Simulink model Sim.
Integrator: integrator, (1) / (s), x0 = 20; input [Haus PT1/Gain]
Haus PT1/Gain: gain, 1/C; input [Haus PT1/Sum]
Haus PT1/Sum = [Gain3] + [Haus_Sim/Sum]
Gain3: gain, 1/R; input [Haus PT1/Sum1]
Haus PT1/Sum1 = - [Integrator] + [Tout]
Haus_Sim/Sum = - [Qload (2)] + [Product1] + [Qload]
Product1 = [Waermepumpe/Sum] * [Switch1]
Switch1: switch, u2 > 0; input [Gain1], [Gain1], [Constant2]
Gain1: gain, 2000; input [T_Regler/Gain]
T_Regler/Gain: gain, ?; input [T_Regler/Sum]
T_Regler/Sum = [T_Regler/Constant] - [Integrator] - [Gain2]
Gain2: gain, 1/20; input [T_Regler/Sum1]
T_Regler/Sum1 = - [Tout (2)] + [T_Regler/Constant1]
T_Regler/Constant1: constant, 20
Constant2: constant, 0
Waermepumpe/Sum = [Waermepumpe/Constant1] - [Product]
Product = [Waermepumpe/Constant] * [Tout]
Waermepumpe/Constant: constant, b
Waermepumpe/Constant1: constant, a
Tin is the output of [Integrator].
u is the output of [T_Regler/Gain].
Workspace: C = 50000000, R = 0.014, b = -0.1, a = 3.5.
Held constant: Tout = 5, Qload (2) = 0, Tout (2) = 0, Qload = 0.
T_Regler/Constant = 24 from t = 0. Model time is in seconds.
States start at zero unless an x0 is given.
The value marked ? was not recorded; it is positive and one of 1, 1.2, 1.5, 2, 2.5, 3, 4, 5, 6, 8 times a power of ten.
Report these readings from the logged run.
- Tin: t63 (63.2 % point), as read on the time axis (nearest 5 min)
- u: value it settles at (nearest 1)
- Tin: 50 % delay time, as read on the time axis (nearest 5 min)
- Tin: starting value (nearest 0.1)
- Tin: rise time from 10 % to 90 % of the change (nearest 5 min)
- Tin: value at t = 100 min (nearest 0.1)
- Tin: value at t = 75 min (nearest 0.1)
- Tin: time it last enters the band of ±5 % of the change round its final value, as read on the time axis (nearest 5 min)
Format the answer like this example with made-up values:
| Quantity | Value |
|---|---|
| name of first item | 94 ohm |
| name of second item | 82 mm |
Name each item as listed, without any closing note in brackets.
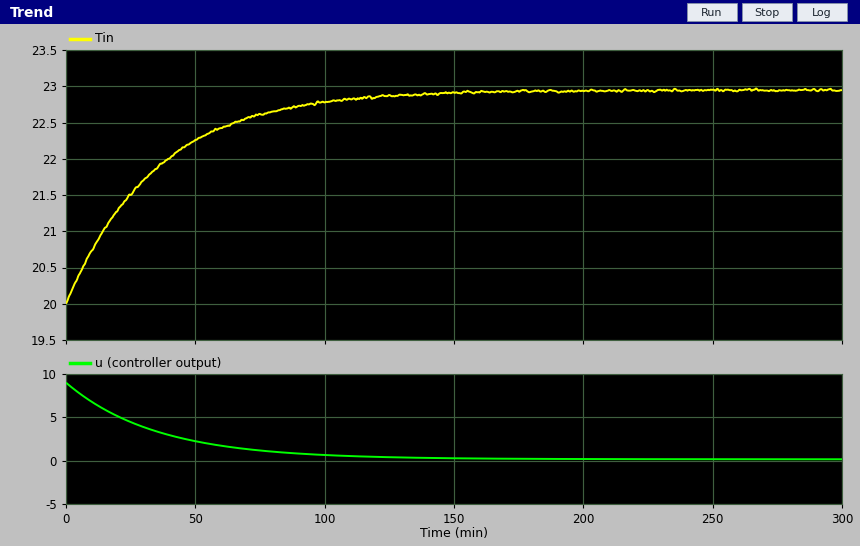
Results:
| Quantity | Value |
|---|---|
| Tin: t63 (63.2 % point), as read on the time axis | 35 min |
| u: value it settles at | 0 |
| Tin: 50 % delay time, as read on the time axis | 25 min |
| Tin: starting value | 20.0 |
| Tin: rise time from 10 % to 90 % of the change | 75 min |
| Tin: value at t = 100 min | 22.8 |
| Tin: value at t = 75 min | 22.6 |
| Tin: time it last enters the band of ±5 % of the change round its final value, as read on the time axis | 105 min |
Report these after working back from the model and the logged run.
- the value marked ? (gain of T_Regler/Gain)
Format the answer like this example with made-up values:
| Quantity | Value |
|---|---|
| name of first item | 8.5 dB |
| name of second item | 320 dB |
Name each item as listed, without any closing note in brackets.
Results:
| Quantity | Value |
|---|---|
| the value marked ? | 3 |
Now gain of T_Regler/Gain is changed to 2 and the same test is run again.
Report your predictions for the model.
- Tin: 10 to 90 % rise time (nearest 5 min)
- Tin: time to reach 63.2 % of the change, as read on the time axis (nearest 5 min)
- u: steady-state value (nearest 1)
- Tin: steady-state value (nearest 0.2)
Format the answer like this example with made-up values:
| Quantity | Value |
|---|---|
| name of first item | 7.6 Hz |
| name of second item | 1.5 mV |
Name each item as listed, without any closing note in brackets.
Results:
| Quantity | Value |
|---|---|
| Tin: 10 to 90 % rise time | 115 min |
| Tin: time to reach 63.2 % of the change, as read on the time axis | 50 min |
| u: steady-state value | 0 |
| Tin: steady-state value | 23.0 |
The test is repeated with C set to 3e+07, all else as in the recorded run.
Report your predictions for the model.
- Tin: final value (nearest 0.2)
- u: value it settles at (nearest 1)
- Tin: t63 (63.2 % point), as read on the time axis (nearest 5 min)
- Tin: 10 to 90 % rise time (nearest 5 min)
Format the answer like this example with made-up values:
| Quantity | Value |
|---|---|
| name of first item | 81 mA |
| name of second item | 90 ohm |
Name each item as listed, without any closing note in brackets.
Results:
| Quantity | Value |
|---|---|
| Tin: final value | 23.0 |
| u: value it settles at | 0 |
| Tin: t63 (63.2 % point), as read on the time axis | 20 min |
| Tin: 10 to 90 % rise time | 45 min |
